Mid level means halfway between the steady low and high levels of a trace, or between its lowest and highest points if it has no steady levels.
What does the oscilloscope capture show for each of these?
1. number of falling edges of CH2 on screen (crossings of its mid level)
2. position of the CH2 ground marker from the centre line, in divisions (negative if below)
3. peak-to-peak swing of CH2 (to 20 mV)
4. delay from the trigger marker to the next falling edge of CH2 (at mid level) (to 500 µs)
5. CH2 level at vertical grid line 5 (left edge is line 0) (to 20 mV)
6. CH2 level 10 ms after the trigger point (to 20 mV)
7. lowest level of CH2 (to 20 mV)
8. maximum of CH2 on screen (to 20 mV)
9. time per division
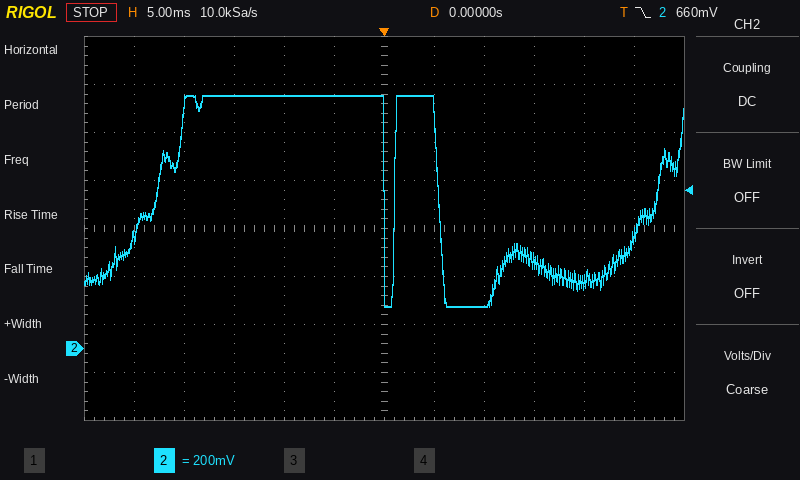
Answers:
2
-2.5 div
880 mV
5.5 ms
1.06 V
180 mV
180 mV
1.06 V
5 ms
